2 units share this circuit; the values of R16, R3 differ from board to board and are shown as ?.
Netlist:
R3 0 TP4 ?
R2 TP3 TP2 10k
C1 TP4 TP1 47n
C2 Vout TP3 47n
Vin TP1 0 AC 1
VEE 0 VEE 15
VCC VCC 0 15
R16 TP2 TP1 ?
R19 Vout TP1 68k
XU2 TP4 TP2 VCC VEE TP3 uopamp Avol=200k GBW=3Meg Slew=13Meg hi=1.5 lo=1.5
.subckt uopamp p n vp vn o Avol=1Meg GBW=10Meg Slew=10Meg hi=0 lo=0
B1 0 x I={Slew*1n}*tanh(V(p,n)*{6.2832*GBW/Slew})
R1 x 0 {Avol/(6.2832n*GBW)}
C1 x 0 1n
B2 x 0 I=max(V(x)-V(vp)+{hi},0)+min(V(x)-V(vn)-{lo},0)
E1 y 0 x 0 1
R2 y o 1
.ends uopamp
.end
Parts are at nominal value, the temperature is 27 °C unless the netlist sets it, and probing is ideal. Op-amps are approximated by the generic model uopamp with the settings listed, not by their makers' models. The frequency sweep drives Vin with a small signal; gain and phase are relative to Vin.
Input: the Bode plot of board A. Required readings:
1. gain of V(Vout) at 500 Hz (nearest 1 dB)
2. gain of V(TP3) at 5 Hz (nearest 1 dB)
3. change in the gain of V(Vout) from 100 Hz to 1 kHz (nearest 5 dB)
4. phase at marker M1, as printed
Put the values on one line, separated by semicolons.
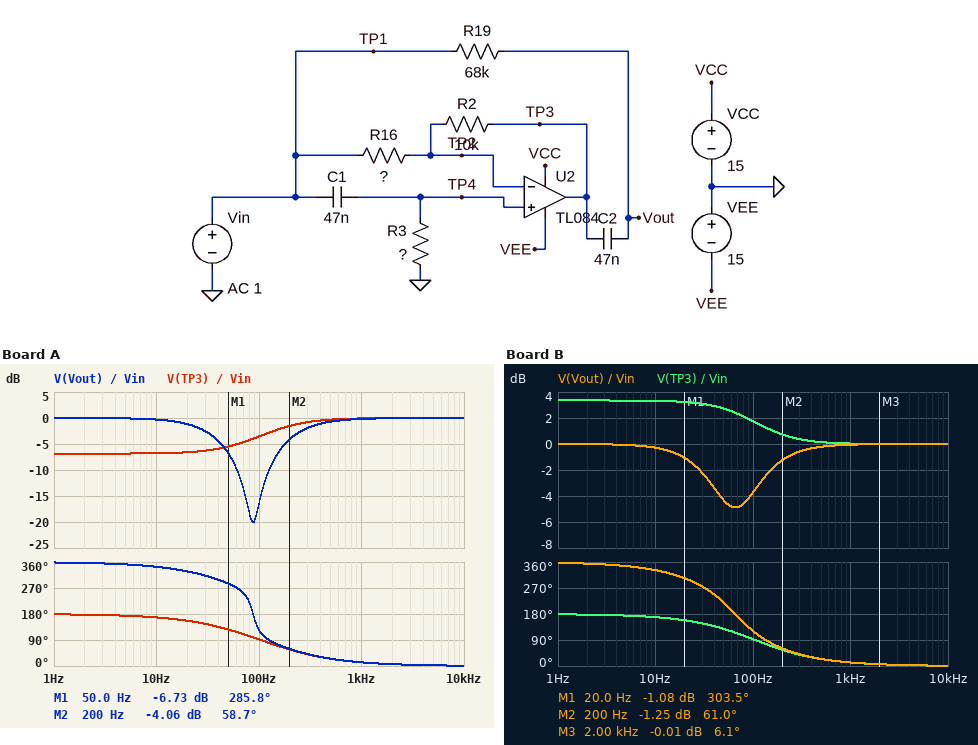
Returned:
-1 dB; -7 dB; 15 dB; 285.8 deg
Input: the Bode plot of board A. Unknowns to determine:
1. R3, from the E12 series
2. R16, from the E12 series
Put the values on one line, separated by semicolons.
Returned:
22 kΩ; 22 kΩ
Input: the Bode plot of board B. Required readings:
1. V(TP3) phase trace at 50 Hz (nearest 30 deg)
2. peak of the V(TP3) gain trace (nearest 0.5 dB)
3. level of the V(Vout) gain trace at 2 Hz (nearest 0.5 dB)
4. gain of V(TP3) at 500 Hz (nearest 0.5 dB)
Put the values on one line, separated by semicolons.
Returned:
120 deg; 3.5 dB; 0 dB; 0 dB
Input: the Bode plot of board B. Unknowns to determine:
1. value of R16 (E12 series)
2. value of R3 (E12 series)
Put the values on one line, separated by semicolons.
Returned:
6.8 kΩ; 39 kΩ
